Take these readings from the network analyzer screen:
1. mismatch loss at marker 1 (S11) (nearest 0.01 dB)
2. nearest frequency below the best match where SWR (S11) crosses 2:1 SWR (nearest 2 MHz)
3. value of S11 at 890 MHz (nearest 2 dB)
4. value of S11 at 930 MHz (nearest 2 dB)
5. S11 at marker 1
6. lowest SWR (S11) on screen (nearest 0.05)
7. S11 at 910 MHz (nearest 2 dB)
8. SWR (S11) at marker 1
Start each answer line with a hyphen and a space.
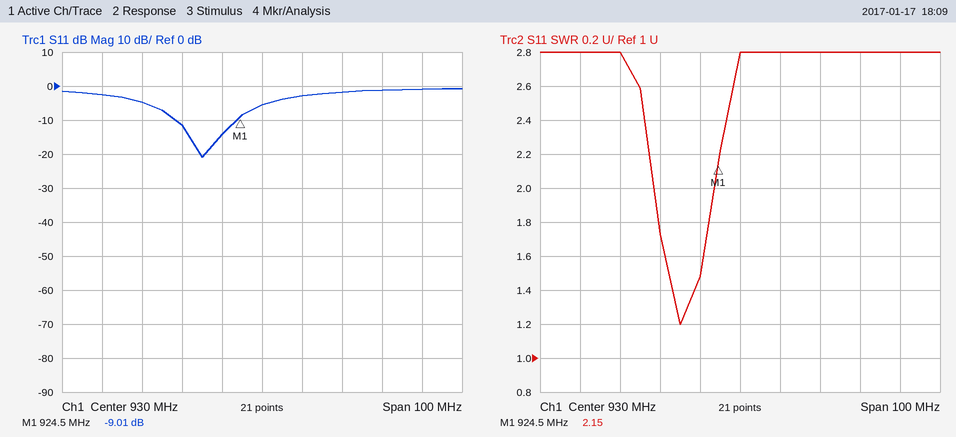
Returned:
- 0.58 dB
- 908 MHz
- -2 dB
- -6 dB
- -9.01 dB
- 1.20
- -12 dB
- 2.15
